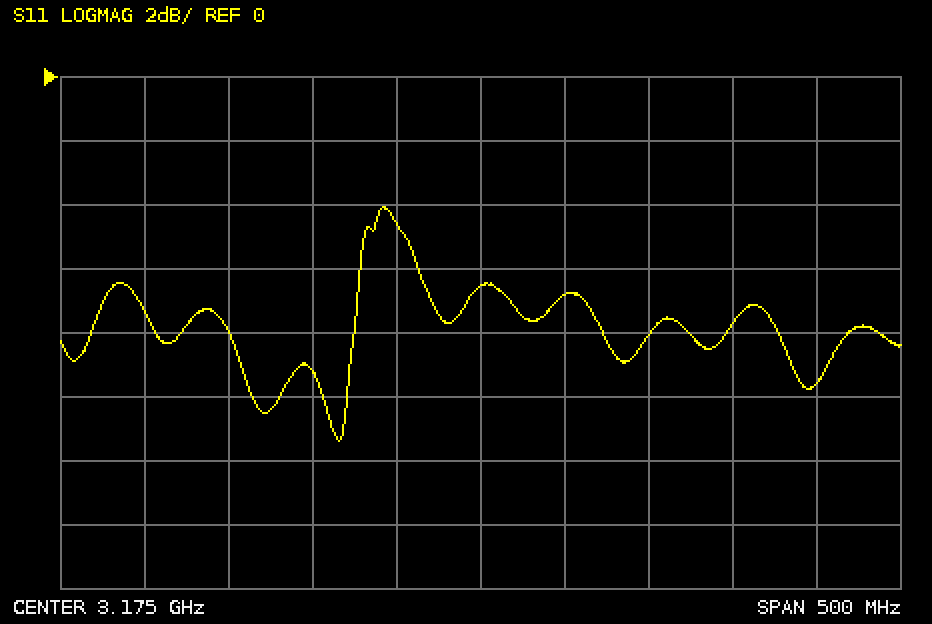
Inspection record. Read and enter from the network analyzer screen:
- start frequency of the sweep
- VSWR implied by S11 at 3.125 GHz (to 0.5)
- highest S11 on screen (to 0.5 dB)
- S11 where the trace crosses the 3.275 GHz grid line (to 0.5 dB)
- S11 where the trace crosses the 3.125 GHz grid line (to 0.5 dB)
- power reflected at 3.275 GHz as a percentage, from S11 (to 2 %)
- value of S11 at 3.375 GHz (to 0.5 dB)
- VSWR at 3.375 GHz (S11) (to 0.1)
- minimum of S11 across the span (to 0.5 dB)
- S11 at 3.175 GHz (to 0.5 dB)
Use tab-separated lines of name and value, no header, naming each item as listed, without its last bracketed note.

start frequency of the sweep	2.925 GHz
VSWR implied by S11 at 3.125 GHz	4.0
highest S11 on screen	-4.0 dB
S11 where the trace crosses the 3.275 GHz grid line	-8.0 dB
S11 where the trace crosses the 3.125 GHz grid line	-4.5 dB
power reflected at 3.275 GHz as a percentage, from S11	16 %
value of S11 at 3.375 GHz	-9.5 dB
VSWR at 3.375 GHz (S11)	2.0
minimum of S11 across the span	-11.5 dB
S11 at 3.175 GHz	-6.5 dB
